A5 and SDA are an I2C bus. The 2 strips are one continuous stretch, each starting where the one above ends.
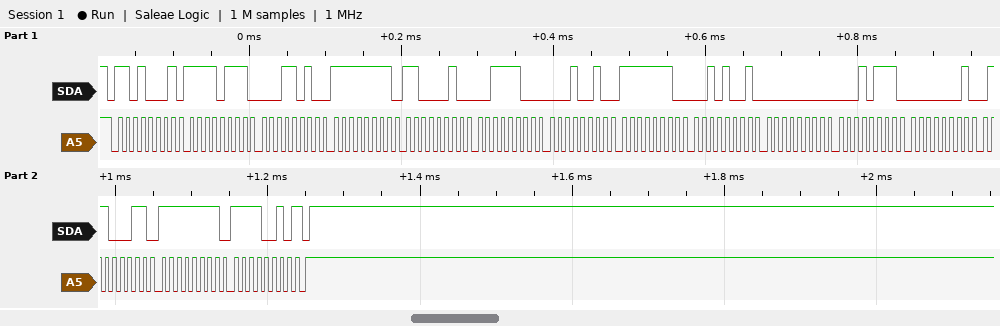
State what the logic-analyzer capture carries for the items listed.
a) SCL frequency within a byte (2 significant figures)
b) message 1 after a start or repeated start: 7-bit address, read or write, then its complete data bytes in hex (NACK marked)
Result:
100 kHz
0x68 read: F7 1A FF C2 3C 12 FE 29 00 17 01 63 FF F2 NACK
